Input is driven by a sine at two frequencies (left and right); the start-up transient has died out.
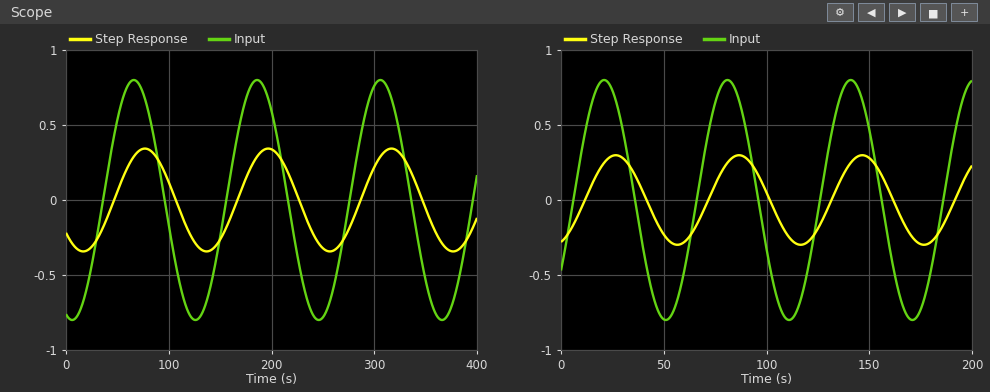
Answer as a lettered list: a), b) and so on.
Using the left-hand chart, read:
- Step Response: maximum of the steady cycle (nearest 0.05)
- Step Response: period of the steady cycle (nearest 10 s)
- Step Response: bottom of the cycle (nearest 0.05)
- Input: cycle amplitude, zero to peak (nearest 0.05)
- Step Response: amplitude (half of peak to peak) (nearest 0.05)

a) 0.35
b) 120 s
c) -0.35
d) 0.80
e) 0.35
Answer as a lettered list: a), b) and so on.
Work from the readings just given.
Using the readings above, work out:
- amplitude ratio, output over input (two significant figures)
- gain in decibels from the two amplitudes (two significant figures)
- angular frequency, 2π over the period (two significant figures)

a) 0.44
b) -7.2 dB
c) 0.052 rad/s
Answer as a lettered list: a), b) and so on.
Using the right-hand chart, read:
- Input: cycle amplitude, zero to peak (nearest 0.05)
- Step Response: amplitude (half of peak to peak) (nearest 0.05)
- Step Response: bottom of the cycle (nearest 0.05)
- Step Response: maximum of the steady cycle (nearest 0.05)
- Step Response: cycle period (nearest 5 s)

a) 0.80
b) 0.30
c) -0.30
d) 0.30
e) 60 s
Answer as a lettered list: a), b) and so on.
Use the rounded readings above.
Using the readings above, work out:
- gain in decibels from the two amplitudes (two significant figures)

a) -8.5 dB
